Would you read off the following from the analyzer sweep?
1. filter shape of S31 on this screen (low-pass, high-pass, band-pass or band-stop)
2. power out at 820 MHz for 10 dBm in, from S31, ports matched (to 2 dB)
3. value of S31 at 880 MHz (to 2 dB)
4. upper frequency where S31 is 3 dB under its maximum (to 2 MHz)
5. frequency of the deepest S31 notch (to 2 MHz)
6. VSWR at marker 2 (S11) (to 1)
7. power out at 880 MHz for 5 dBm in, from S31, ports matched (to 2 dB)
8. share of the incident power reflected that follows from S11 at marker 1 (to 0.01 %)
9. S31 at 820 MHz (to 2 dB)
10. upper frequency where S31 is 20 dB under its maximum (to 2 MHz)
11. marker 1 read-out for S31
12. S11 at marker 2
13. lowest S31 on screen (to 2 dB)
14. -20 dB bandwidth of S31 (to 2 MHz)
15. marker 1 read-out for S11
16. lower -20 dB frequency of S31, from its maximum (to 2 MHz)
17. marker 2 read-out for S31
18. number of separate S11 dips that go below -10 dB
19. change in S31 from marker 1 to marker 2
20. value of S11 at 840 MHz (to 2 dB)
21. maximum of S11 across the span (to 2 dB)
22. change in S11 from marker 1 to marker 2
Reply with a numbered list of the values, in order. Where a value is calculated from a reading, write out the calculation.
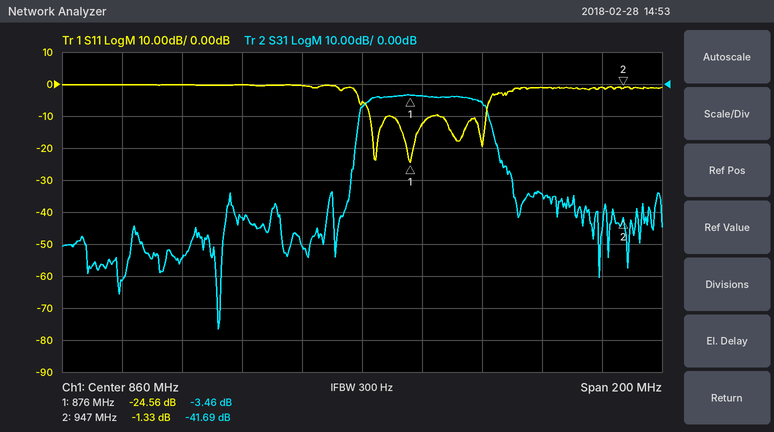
1. band-pass
2. 10 dBm + (-42 dB) = -32 dBm
3. -4 dB
4. 900 MHz
5. 812 MHz
6. (1 + 0.8580)/(1 − 0.8580) ≈ 13
7. 5 dBm + (-4 dB) = 2 dBm
8. 10^(-24.56/10) ≈ 0.35 %
9. -42 dB
10. 906 MHz
11. -3.46 dB
12. -1.33 dB
13. -76 dB
14. 906 MHz − 858 MHz = 48 MHz
15. -24.56 dB
16. 858 MHz
17. -41.69 dB
18. 4
19. -41.69 − (-3.46) = -38.23 dB
20. 0 dB
21. 0 dB
22. -1.33 − (-24.56) = 23.23 dB
